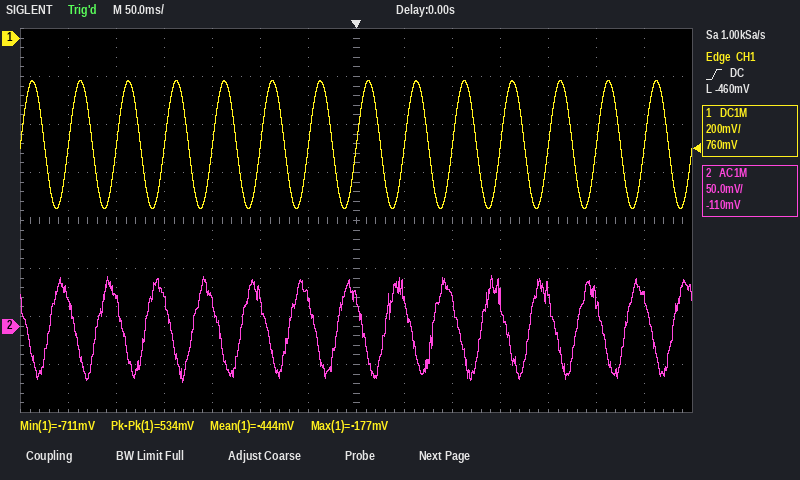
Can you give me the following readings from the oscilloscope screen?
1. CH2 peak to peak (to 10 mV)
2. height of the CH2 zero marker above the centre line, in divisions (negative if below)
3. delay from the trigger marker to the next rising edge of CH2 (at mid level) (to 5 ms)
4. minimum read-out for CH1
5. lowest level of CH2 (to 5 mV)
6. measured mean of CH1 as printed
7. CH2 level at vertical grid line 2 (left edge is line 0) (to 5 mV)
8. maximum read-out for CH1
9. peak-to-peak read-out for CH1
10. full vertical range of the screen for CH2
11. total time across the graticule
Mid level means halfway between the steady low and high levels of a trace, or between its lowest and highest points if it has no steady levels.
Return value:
110 mV
-2.2 div
30 ms
-711 mV
-60 mV
-444 mV
30 mV
-177 mV
534 mV
400 mV
700 ms
